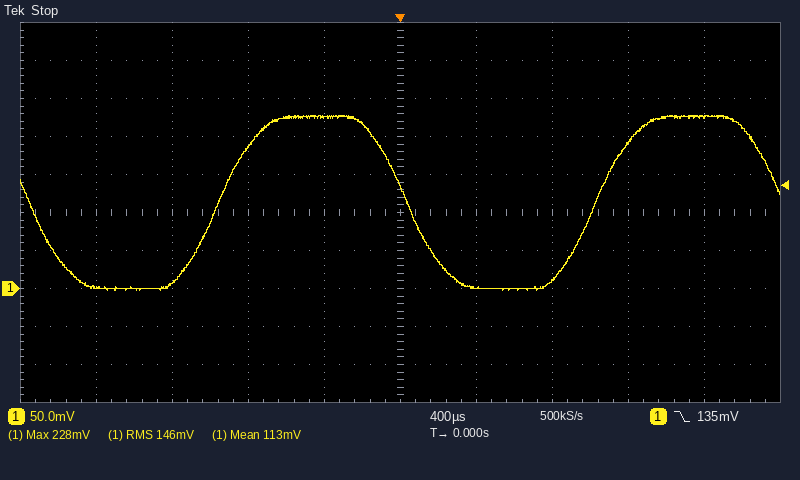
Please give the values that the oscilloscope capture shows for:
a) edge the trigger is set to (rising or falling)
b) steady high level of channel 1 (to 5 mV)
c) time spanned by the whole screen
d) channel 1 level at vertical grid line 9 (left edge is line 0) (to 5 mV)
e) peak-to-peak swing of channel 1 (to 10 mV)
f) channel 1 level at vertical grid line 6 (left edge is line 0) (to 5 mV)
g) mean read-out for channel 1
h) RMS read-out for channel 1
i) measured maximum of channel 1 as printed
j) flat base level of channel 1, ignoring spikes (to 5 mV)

falling
225 mV
4 ms
225 mV
230 mV
0 mV
113 mV
146 mV
228 mV
0 mV
